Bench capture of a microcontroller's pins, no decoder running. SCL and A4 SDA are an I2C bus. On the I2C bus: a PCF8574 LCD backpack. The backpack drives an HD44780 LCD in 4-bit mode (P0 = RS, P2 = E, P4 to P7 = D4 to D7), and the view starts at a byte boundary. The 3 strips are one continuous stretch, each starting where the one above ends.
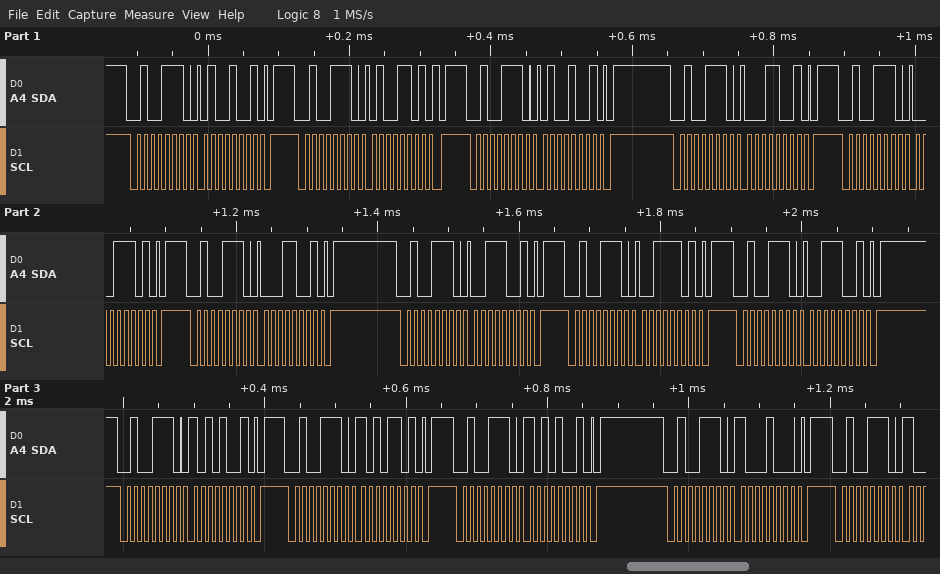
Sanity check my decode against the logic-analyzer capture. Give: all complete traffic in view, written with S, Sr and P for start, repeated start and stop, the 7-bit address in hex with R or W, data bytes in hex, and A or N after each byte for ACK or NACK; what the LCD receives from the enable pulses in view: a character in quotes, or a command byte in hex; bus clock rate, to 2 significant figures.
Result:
S 27W A 49 A P S 27W A 4D A P S 27W A 49 A P S 27W A 19 A P S 27W A 1D A P S 27W A 19 A P S 27W A 39 A P S 27W A 3D A P S 27W A 39 A P S 27W A A9 A P S 27W A AD A P S 27W A A9 A P S 27W A 88 A P S 27W A
'A' ':'
100 kHz
